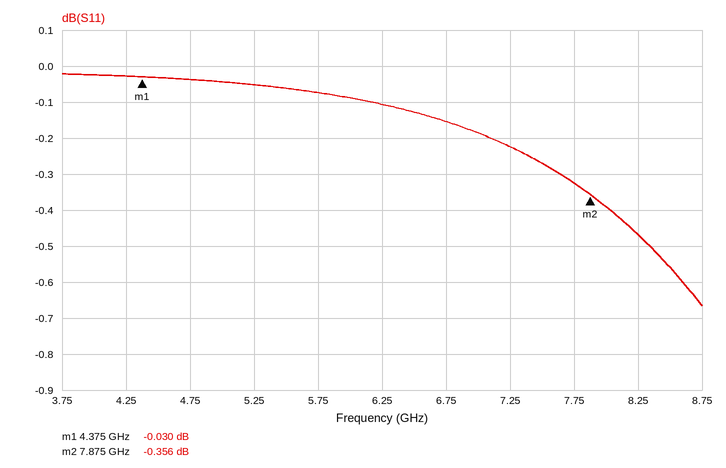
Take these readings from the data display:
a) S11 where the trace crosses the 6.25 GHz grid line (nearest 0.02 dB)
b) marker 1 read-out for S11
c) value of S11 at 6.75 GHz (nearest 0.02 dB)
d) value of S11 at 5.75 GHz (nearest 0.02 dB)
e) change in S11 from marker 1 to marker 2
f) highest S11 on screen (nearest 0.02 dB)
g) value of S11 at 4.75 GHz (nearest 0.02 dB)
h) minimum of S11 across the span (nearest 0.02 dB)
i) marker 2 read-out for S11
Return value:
-0.10 dB
-0.030 dB
-0.16 dB
-0.08 dB
-0.326 dB
-0.02 dB
-0.04 dB
-0.66 dB
-0.356 dB
